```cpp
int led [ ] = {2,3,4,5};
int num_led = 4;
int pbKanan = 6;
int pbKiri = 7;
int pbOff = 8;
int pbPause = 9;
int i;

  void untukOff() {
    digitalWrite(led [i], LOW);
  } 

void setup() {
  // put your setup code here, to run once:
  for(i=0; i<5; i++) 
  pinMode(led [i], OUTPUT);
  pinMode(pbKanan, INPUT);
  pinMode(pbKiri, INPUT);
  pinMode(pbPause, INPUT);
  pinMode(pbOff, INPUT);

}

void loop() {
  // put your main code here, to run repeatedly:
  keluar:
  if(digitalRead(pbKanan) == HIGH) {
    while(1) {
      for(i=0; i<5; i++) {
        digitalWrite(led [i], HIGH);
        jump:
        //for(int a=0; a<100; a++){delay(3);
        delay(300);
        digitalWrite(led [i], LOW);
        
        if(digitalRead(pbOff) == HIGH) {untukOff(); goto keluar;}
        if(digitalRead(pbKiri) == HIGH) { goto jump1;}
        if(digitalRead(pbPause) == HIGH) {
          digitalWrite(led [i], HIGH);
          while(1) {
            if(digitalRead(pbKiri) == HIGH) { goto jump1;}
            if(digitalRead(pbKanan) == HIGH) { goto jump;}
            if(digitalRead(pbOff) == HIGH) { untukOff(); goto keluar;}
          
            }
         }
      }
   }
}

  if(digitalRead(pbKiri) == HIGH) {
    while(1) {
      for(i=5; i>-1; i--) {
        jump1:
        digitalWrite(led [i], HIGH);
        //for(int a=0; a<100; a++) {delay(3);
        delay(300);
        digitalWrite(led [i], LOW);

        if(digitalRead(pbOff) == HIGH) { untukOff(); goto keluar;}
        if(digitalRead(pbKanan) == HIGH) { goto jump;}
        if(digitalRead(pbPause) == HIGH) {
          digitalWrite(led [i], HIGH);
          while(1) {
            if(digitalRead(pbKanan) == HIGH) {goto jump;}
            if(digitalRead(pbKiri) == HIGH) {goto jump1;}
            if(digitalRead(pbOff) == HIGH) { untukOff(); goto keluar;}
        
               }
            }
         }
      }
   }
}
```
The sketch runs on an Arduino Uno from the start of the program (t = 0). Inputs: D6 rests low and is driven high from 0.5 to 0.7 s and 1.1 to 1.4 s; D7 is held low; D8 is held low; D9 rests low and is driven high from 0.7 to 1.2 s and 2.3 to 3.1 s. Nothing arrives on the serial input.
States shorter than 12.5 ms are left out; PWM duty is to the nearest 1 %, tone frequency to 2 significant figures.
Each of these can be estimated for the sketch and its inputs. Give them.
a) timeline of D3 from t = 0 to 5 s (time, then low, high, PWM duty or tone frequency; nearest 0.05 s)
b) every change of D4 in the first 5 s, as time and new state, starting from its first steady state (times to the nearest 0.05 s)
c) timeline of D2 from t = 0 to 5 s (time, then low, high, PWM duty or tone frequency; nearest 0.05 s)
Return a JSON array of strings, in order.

["0 s low; 1.4 s high; 1.7 s low", "0 s low; 1.7 s high; 2 s low", "0 s low; 0.5 s high; 1.4 s low"]
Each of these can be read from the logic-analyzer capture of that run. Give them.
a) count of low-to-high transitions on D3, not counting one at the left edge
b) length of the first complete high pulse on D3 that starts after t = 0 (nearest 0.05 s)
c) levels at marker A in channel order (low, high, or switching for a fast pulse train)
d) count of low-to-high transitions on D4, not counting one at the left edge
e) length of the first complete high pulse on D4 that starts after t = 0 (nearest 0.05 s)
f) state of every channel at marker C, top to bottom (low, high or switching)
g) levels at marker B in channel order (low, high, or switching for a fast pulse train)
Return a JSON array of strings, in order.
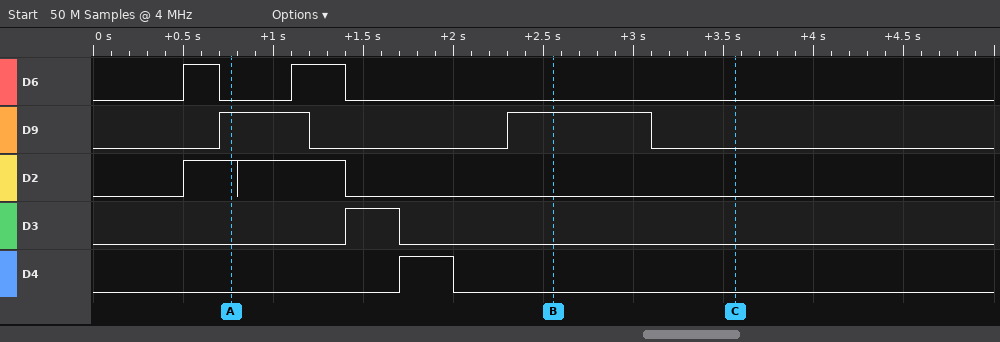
["1", "0.30 s", "D6 low, D9 high, D2 high, D3 low, D4 low", "1", "0.30 s", "D6 low, D9 low, D2 low, D3 low, D4 low", "D6 low, D9 high, D2 low, D3 low, D4 low"]
